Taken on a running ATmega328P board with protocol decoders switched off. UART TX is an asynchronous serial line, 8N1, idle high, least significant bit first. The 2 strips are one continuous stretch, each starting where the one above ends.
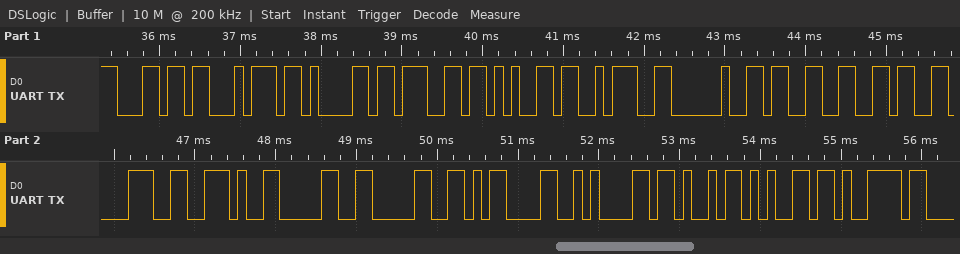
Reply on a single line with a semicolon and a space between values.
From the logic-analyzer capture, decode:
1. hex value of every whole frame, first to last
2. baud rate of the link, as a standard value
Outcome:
6C 74 61 67 65 3A 20 33 36 38 2E 30 30 0D 0A 4B 65 79; 9600 baud
